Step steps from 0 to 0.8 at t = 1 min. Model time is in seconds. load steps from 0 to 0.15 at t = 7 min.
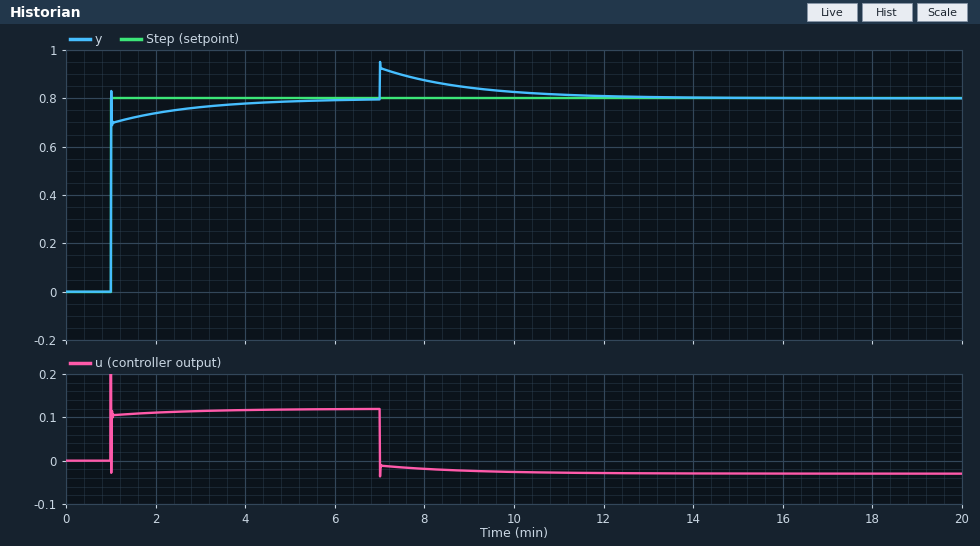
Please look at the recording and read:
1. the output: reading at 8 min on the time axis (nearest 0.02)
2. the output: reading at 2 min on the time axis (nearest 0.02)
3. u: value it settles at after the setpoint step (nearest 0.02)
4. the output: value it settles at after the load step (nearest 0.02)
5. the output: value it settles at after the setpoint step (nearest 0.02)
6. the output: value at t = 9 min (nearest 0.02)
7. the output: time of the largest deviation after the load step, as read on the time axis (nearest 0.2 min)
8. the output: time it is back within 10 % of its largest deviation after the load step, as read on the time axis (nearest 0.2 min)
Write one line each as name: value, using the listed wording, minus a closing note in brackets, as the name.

the output: reading at 8 min on the time axis: 0.88
the output: reading at 2 min on the time axis: 0.74
u: value it settles at after the setpoint step: 0.12
the output: value it settles at after the load step: 0.80
the output: value it settles at after the setpoint step: 0.80
the output: value at t = 9 min: 0.84
the output: time of the largest deviation after the load step, as read on the time axis: 7.0 min
the output: time it is back within 10 % of its largest deviation after the load step, as read on the time axis: 11.0 min
